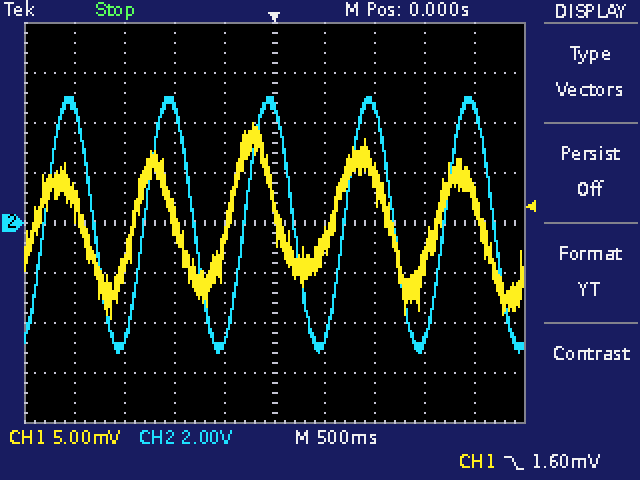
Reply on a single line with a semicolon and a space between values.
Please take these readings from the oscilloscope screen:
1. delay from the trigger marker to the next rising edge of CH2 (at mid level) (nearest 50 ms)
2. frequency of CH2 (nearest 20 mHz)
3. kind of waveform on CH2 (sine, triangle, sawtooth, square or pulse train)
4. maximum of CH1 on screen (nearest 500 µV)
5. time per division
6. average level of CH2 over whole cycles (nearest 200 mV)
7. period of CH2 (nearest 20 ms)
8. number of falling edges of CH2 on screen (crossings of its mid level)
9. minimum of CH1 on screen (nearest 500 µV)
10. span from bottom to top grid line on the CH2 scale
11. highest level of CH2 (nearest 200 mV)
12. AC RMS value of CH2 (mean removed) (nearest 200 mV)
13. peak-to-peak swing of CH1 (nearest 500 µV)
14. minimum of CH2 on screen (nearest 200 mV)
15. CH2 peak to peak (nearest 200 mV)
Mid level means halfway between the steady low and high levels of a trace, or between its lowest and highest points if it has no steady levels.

700 ms; 1.00 Hz; sine; 10.0 mV; 500 ms; 0.0 V; 1.00 s; 5; -9.5 mV; 16 V; 5.0 V; 3.6 V; 19.5 mV; -5.2 V; 10.2 V
